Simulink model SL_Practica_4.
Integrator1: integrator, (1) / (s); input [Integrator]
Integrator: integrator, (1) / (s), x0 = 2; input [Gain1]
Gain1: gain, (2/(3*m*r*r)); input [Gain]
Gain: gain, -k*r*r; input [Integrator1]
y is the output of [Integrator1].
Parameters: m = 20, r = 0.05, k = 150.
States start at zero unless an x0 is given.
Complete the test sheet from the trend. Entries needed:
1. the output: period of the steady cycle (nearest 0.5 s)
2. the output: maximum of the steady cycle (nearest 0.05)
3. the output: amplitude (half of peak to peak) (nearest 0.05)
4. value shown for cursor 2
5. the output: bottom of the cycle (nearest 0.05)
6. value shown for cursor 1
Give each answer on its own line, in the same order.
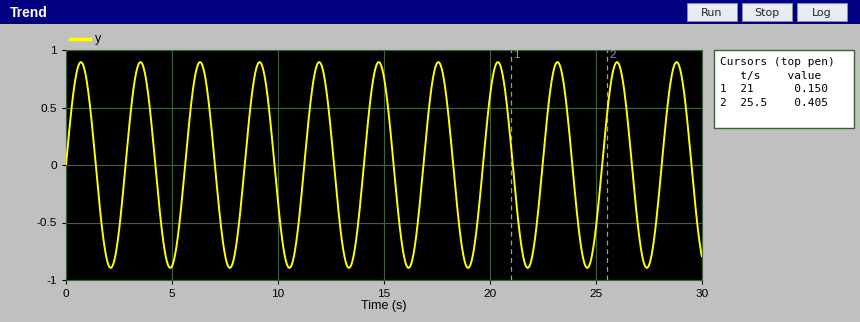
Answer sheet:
3.0 s
0.90
0.90
0.405
-0.90
0.150
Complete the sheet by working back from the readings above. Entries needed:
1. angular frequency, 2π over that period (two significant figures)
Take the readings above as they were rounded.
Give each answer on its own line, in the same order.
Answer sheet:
2.1 rad/s
